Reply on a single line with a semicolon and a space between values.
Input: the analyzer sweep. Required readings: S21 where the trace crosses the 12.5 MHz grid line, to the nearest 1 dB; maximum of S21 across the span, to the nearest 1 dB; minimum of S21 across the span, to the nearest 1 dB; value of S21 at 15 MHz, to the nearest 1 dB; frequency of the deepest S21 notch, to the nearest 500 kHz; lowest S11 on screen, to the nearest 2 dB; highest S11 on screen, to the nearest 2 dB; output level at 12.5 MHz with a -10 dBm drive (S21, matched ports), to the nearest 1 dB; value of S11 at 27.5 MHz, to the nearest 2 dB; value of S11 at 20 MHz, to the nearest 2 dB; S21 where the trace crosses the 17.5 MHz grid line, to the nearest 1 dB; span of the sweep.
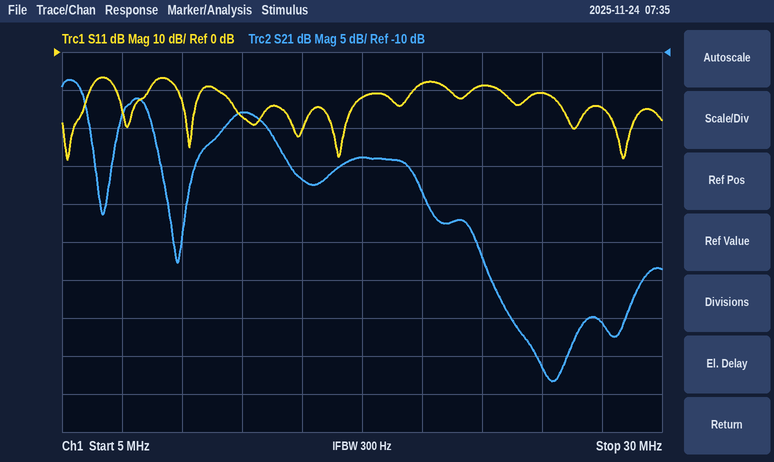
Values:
-18 dB; -14 dB; -53 dB; -27 dB; 25.5 MHz; -28 dB; -6 dB; -28 dBm; -14 dB; -8 dB; -24 dB; 25 MHz
